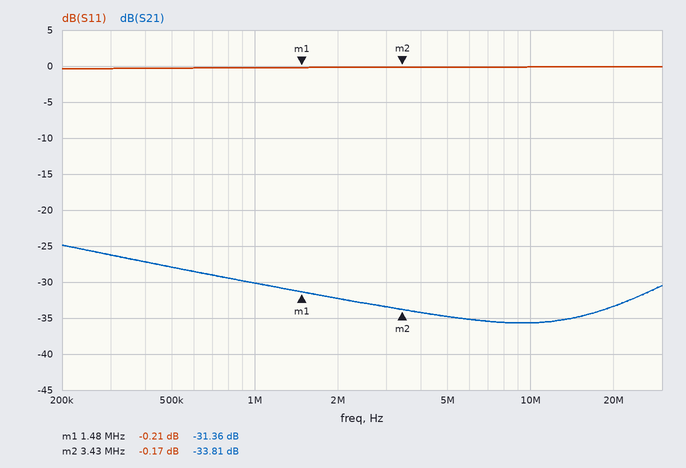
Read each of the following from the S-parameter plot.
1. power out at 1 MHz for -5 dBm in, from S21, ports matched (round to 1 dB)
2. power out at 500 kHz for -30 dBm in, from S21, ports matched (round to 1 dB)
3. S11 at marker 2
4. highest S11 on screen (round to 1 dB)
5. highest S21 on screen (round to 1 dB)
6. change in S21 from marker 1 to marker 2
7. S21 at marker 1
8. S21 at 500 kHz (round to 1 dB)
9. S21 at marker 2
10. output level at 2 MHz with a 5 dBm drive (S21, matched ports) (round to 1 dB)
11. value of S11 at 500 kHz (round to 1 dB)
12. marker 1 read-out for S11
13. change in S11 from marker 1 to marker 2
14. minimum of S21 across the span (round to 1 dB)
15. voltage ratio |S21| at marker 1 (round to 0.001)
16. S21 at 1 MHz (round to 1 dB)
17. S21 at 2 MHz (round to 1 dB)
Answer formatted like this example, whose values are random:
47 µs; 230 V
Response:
-35 dBm; -58 dBm; -0.17 dB; 0 dB; -25 dB; -2.45 dB; -31.36 dB; -28 dB; -33.81 dB; -27 dBm; 0 dB; -0.21 dB; 0.04 dB; -36 dB; 0.027; -30 dB; -32 dB
